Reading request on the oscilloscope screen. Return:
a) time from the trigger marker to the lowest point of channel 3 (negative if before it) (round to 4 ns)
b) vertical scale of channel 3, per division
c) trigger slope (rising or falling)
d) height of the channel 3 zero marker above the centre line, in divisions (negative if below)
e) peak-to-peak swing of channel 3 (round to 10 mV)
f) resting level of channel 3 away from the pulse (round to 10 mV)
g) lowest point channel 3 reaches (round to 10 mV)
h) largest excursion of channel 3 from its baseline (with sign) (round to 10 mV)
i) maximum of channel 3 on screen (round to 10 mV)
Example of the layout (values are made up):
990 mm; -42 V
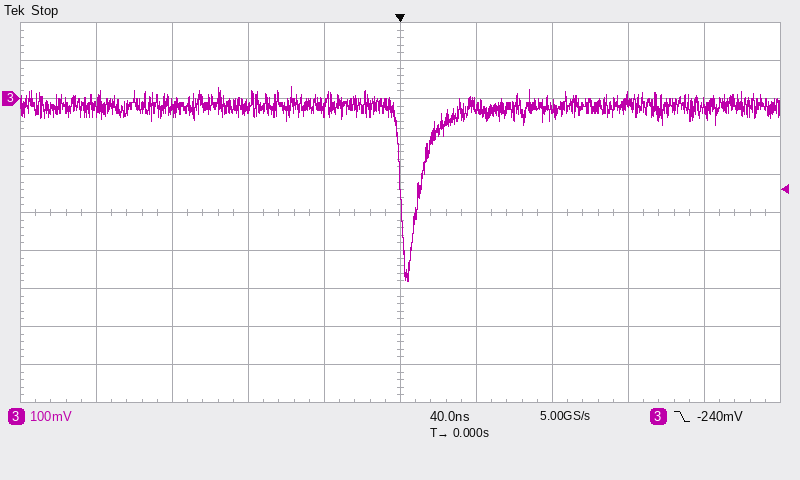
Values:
+4 ns; 100 mV; falling; +3.0 div; 510 mV; -20 mV; -480 mV; -460 mV; 30 mV
